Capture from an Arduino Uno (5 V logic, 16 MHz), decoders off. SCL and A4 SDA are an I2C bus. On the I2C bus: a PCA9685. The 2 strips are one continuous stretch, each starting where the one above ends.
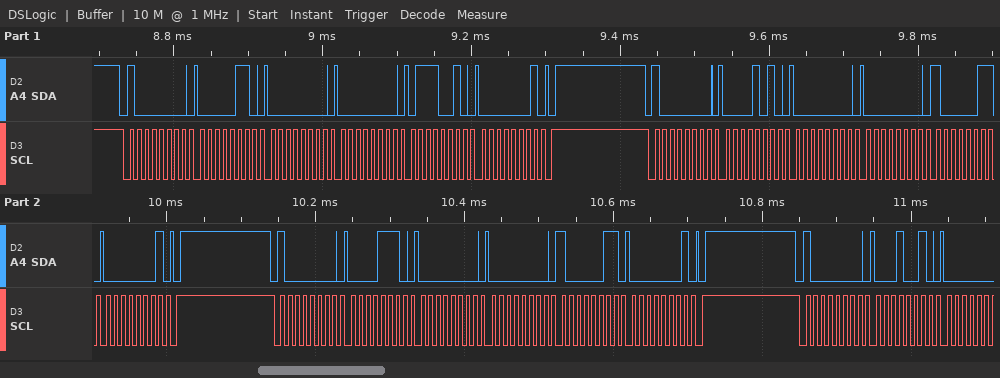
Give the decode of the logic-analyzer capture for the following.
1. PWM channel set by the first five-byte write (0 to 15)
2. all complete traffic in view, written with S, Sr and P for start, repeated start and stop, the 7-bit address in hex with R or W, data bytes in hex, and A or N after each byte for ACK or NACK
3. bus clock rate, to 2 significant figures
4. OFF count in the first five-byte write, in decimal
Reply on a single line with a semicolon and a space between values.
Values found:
0; S 40W A 06 A 00 A 00 A 72 A 01 A P S 40W A 0A A 00 A 00 A 83 A 01 A P S 40W A 0E A 00 A 00 A 83 A 01 A P S 40W A 12 A; 100 kHz; 370
